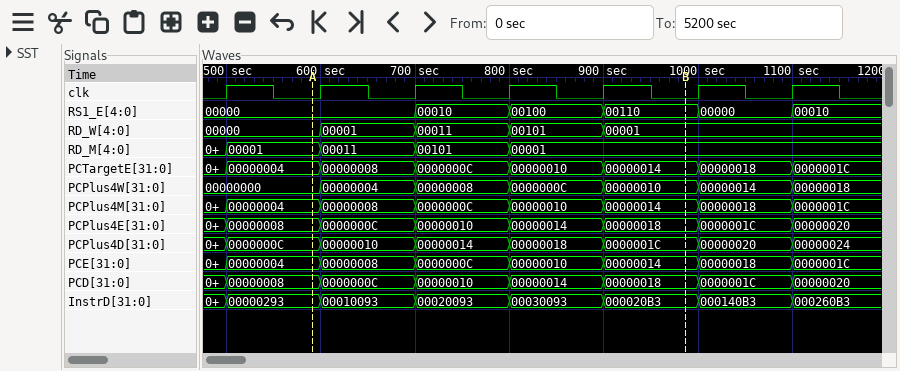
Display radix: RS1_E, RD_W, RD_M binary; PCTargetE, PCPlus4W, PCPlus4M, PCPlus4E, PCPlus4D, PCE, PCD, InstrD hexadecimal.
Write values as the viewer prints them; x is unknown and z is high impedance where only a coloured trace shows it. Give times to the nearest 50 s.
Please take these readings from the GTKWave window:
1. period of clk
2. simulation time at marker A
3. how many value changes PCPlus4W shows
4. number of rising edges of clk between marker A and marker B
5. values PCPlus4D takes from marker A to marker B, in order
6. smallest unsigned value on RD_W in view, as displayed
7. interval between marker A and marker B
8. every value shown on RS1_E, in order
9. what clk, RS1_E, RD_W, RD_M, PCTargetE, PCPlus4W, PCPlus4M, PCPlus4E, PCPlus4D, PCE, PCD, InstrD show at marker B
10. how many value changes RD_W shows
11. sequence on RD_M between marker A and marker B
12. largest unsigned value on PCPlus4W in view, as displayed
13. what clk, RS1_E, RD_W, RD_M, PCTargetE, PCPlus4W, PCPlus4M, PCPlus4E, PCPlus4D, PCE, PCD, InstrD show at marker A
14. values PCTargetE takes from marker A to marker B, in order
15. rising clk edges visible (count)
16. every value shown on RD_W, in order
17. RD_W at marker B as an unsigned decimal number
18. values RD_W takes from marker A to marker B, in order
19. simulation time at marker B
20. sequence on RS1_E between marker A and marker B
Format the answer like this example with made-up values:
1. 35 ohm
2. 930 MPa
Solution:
1. 100 s
2. 600 s
3. 6
4. 4
5. 0000000C, 00000010, 00000014, 00000018, 0000001C
6. 00000
7. 400 s
8. 00000, 00010, 00100, 00110, 00000, 00010
9. clk=0, RS1_E=00110, RD_W=00001, RD_M=00001, PCTargetE=00000014, PCPlus4W=00000010, PCPlus4M=00000014, PCPlus4E=00000018, PCPlus4D=0000001C, PCE=00000014, PCD=00000018, InstrD=000020B3
10. 4
11. 00001, 00011, 00101, 00001
12. 00000018
13. clk=0, RS1_E=00000, RD_W=00000, RD_M=00001, PCTargetE=00000004, PCPlus4W=00000000, PCPlus4M=00000004, PCPlus4E=00000008, PCPlus4D=0000000C, PCE=00000004, PCD=00000008, InstrD=00000293
14. 00000004, 00000008, 0000000C, 00000010, 00000014
15. 7
16. 00000, 00001, 00011, 00101, 00001
17. 1
18. 00000, 00001, 00011, 00101, 00001
19. 1000 s
20. 00000, 00010, 00100, 00110
